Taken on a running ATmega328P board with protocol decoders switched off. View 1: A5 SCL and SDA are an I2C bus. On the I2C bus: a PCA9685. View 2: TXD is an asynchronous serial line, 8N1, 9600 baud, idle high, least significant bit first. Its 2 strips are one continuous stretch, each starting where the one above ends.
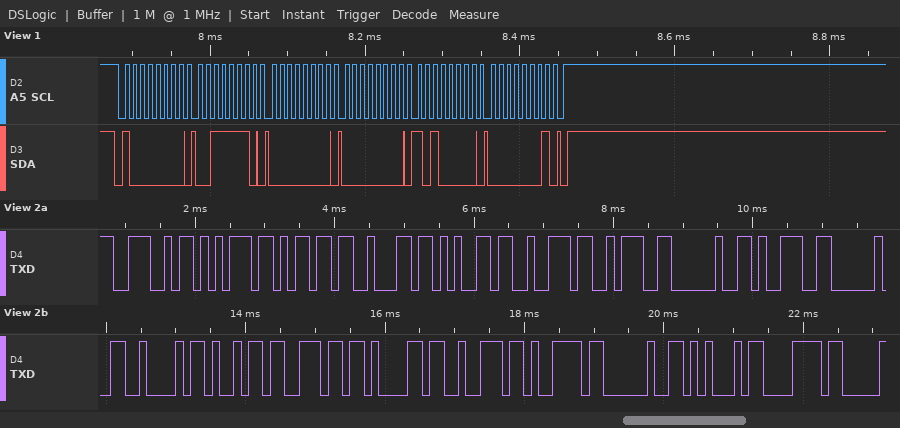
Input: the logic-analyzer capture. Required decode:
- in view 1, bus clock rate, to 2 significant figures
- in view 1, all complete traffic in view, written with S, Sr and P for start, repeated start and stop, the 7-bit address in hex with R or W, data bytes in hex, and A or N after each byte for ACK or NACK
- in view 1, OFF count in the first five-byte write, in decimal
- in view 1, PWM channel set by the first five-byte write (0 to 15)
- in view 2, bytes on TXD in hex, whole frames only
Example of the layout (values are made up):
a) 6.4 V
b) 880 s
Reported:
a) 100 kHz
b) S 40W A 3E A 00 A 00 A A0 A 01 A P
c) 416
d) 14
e) 4E 75 6D 62 65 72 3A 20 39 20 42 69 6E 61 72 79 20 45 78
